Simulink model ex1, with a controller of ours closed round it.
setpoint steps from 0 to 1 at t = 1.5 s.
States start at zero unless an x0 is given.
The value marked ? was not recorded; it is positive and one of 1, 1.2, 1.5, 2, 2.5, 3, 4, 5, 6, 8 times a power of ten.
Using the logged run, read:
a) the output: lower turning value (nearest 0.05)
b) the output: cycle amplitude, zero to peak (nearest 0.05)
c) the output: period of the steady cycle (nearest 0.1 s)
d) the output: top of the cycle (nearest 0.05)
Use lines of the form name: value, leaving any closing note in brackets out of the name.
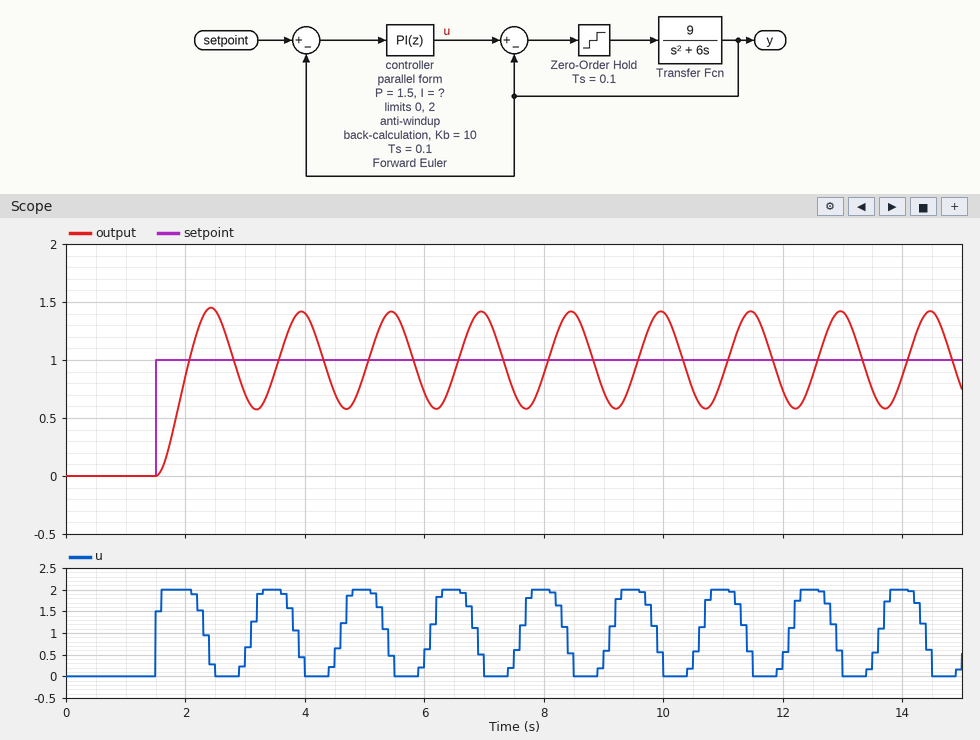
the output: lower turning value: 0.60
the output: cycle amplitude, zero to peak: 0.40
the output: period of the steady cycle: 1.5 s
the output: top of the cycle: 1.40
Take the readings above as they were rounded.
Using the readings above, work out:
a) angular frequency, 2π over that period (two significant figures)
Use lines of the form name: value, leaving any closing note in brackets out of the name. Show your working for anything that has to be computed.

angular frequency, 2π over that period: 2π / 1.5 = 4.2 rad/s
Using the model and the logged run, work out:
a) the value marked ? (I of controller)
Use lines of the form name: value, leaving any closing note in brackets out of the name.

the value marked ?: 15
